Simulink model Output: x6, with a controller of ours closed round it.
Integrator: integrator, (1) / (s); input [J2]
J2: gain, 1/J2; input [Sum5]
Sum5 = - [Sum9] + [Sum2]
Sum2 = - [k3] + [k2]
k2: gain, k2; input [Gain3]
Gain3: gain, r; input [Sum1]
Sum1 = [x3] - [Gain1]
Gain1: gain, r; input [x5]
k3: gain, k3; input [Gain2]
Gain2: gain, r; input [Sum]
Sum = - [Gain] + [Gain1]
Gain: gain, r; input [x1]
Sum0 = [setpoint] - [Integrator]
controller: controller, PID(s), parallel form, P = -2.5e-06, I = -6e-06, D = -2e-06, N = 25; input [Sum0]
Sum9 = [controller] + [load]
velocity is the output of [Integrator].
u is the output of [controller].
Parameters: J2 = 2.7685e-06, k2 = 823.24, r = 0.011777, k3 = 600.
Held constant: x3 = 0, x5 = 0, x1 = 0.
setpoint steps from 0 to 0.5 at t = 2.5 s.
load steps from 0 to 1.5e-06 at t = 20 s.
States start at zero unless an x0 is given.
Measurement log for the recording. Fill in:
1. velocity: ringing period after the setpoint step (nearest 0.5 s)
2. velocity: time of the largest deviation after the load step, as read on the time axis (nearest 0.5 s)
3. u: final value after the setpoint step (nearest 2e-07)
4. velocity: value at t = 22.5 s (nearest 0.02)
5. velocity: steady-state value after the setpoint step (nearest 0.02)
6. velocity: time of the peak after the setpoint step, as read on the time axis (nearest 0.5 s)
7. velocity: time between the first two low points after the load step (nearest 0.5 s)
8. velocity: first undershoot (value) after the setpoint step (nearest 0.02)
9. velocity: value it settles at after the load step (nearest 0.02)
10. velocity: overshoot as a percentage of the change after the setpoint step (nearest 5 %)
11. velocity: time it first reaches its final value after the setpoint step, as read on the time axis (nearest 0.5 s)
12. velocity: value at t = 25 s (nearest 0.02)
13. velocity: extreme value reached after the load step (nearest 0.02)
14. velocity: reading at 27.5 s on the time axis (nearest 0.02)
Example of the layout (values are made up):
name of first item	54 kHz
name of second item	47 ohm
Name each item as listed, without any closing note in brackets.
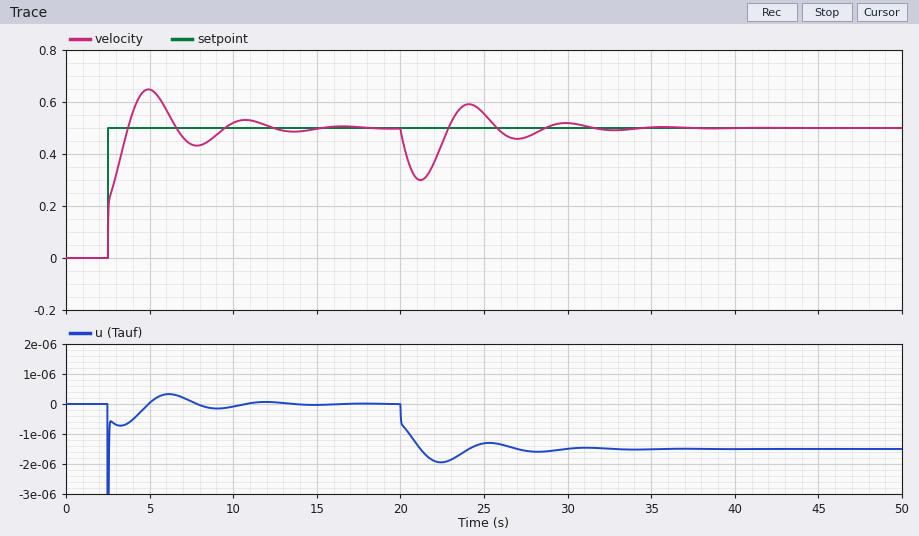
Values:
velocity: ringing period after the setpoint step	6.0 s
velocity: time of the largest deviation after the load step, as read on the time axis	21.0 s
u: final value after the setpoint step	0.0000000
velocity: value at t = 22.5 s	0.44
velocity: steady-state value after the setpoint step	0.50
velocity: time of the peak after the setpoint step, as read on the time axis	5.0 s
velocity: time between the first two low points after the load step	6.0 s
velocity: first undershoot (value) after the setpoint step	0.44
velocity: value it settles at after the load step	0.50
velocity: overshoot as a percentage of the change after the setpoint step	30 %
velocity: time it first reaches its final value after the setpoint step, as read on the time axis	3.5 s
velocity: value at t = 25 s	0.56
velocity: extreme value reached after the load step	0.30
velocity: reading at 27.5 s on the time axis	0.46
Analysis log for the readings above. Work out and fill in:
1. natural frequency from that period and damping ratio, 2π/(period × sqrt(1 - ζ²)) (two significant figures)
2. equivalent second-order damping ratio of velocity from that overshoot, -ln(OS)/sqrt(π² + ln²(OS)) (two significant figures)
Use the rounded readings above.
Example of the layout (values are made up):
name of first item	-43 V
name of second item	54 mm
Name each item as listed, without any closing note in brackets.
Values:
natural frequency from that period and damping ratio, 2π/(period × sqrt(1 - ζ²))	1.1 rad/s
equivalent second-order damping ratio of velocity from that overshoot, -ln(OS)/sqrt(π² + ln²(OS))	0.36
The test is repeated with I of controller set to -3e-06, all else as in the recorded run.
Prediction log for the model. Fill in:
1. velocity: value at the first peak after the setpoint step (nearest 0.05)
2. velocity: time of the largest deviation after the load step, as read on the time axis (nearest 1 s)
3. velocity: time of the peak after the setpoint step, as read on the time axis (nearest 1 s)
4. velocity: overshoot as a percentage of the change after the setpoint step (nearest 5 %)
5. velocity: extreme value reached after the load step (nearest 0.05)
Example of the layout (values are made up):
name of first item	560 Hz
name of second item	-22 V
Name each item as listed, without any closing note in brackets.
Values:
velocity: value at the first peak after the setpoint step	0.60
velocity: time of the largest deviation after the load step, as read on the time axis	22 s
velocity: time of the peak after the setpoint step, as read on the time axis	6 s
velocity: overshoot as a percentage of the change after the setpoint step	25 %
velocity: extreme value reached after the load step	0.25
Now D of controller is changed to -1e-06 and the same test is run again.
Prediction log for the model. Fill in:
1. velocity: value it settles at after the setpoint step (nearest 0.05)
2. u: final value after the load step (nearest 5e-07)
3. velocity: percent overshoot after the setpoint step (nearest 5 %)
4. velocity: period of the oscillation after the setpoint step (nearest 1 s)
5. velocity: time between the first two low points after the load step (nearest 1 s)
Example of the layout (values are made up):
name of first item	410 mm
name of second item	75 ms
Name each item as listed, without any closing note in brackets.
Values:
velocity: value it settles at after the setpoint step	0.50
u: final value after the load step	-0.0000015
velocity: percent overshoot after the setpoint step	35 %
velocity: period of the oscillation after the setpoint step	5 s
velocity: time between the first two low points after the load step	5 s
